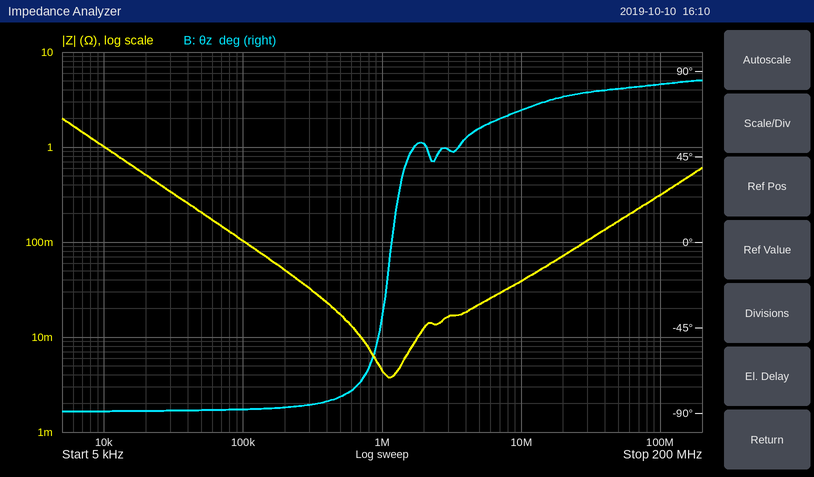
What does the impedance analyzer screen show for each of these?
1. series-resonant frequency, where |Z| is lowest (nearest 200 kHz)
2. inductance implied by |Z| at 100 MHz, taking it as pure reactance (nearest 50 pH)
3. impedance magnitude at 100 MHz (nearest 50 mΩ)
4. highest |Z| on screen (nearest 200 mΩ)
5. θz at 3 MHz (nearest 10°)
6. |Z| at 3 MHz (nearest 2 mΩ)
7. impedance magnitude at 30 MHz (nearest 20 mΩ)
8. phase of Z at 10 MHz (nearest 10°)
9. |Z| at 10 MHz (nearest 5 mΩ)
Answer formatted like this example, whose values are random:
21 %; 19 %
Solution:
1.2 MHz; 500 pH; 300 mΩ; 2.0 Ω; 50°; 16 mΩ; 100 mΩ; 70°; 40 mΩ
